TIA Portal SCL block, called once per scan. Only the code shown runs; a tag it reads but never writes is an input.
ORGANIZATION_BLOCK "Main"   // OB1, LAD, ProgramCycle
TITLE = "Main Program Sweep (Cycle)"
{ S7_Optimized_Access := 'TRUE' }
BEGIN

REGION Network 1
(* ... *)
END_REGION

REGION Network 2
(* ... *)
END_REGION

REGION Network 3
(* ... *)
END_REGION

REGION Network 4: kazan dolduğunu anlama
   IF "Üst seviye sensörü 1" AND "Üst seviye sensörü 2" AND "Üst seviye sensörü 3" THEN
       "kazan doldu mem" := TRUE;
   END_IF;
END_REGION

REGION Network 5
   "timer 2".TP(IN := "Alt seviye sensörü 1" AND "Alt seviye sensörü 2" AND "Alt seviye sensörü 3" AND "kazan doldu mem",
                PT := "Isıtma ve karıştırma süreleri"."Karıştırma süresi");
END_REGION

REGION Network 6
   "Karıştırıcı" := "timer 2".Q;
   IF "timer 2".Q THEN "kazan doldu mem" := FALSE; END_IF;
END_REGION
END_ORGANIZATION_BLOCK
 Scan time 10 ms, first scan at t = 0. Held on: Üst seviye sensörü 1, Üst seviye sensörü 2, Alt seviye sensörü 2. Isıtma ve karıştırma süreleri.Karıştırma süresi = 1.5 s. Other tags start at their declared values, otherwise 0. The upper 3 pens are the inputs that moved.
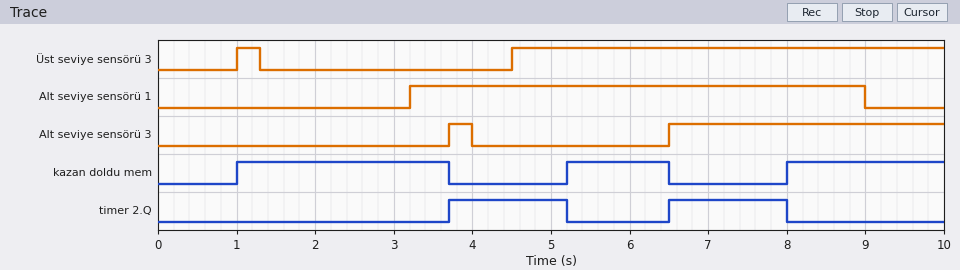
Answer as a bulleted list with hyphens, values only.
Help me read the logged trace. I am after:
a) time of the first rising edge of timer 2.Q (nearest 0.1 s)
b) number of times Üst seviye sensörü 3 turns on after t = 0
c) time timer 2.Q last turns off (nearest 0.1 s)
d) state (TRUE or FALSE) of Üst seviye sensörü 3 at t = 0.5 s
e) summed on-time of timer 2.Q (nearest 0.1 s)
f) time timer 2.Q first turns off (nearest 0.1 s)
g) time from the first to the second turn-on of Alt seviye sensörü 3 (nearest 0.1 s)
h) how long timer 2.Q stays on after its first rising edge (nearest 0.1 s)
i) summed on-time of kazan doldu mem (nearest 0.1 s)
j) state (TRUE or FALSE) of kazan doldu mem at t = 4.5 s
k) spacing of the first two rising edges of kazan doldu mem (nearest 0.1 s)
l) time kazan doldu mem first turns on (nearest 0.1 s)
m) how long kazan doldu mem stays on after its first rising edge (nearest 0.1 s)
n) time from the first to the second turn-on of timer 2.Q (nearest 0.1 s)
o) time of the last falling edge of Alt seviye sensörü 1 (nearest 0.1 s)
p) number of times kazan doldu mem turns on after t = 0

- 3.7 s
- 2
- 8.0 s
- FALSE
- 3.0 s
- 5.2 s
- 2.8 s
- 1.5 s
- 6.0 s
- FALSE
- 4.2 s
- 1.0 s
- 2.7 s
- 2.8 s
- 9.0 s
- 3
